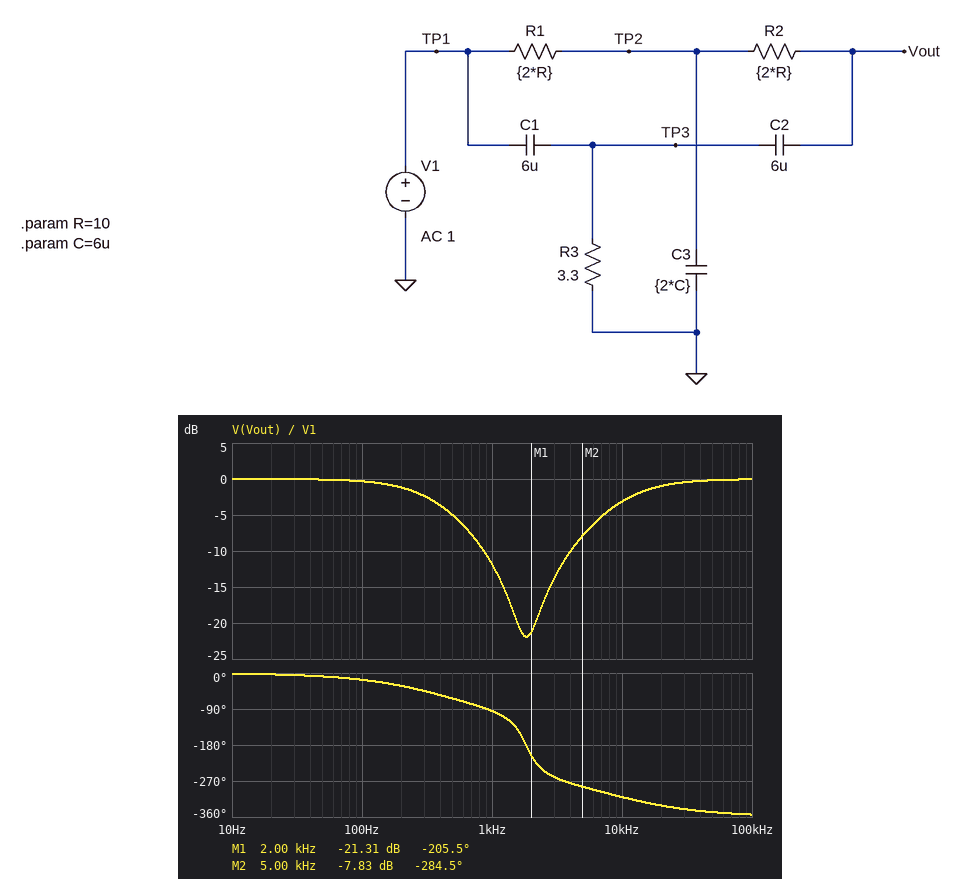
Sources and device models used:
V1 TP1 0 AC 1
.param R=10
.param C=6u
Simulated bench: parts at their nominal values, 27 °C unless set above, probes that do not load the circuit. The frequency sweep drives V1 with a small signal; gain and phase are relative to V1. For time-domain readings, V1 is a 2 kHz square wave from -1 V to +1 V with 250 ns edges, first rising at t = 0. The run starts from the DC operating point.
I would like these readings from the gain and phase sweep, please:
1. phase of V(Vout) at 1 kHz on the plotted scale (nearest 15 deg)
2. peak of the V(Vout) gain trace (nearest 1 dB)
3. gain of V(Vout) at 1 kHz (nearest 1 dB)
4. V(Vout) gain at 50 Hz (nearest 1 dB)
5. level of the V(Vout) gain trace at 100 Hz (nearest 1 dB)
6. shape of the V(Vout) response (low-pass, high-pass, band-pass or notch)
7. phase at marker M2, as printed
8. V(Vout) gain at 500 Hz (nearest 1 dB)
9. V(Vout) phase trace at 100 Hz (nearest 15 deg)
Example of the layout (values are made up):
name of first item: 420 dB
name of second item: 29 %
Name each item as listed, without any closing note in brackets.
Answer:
phase of V(Vout) at 1 kHz on the plotted scale: -90 deg
peak of the V(Vout) gain trace: 0 dB
gain of V(Vout) at 1 kHz: -12 dB
V(Vout) gain at 50 Hz: 0 dB
level of the V(Vout) gain trace at 100 Hz: 0 dB
shape of the V(Vout) response: notch
phase at marker M2, as printed: -284.5 deg
V(Vout) gain at 500 Hz: -5 dB
V(Vout) phase trace at 100 Hz: -15 deg
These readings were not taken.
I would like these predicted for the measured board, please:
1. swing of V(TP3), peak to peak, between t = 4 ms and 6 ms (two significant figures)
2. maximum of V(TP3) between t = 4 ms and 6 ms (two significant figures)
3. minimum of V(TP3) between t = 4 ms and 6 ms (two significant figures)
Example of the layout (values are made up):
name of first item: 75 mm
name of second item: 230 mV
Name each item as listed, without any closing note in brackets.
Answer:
swing of V(TP3), peak to peak, between t = 4 ms and 6 ms: 3.9 V
maximum of V(TP3) between t = 4 ms and 6 ms: 1.9 V
minimum of V(TP3) between t = 4 ms and 6 ms: -1.9 V
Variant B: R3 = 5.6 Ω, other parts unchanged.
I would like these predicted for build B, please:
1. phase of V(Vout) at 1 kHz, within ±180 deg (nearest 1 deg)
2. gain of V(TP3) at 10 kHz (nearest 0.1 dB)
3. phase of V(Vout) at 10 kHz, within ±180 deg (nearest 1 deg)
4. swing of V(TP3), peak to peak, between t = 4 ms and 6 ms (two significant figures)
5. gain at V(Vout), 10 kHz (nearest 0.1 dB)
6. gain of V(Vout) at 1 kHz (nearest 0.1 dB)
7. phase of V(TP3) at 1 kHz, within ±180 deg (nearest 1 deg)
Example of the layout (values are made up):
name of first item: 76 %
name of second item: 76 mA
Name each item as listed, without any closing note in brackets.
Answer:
phase of V(Vout) at 1 kHz, within ±180 deg: -94 deg
gain of V(TP3) at 10 kHz: -1.6 dB
phase of V(Vout) at 10 kHz, within ±180 deg: 38 deg
swing of V(TP3), peak to peak, between t = 4 ms and 6 ms: 3.8 V
gain at V(Vout), 10 kHz: -1.8 dB
gain of V(Vout) at 1 kHz: -13.6 dB
phase of V(TP3) at 1 kHz, within ±180 deg: 55 deg
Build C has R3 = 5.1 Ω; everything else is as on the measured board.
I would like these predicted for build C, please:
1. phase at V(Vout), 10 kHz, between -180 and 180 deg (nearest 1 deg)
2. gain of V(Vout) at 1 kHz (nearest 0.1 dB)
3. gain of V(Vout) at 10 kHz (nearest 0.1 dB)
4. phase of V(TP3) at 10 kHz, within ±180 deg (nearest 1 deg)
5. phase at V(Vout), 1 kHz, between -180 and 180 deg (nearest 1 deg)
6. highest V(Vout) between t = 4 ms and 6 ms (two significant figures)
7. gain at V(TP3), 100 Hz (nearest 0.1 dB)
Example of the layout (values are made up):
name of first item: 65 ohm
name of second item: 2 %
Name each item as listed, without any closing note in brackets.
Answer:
phase at V(Vout), 10 kHz, between -180 and 180 deg: 40 deg
gain of V(Vout) at 1 kHz: -13.2 dB
gain of V(Vout) at 10 kHz: -2.0 dB
phase of V(TP3) at 10 kHz, within ±180 deg: 32 deg
phase at V(Vout), 1 kHz, between -180 and 180 deg: -94 deg
highest V(Vout) between t = 4 ms and 6 ms: 1.8 V
gain at V(TP3), 100 Hz: -28.6 dB
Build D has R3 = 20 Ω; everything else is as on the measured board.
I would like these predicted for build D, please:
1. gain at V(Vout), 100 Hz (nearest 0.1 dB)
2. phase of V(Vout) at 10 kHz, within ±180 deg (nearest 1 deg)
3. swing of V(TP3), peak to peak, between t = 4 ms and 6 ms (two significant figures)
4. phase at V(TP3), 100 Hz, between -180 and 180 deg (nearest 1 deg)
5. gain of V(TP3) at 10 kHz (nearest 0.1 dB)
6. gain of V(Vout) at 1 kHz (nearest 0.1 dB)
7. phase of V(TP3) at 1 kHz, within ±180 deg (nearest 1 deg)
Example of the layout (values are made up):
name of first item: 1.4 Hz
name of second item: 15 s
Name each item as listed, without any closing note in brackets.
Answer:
gain at V(Vout), 100 Hz: -0.5 dB
phase of V(Vout) at 10 kHz, within ±180 deg: 22 deg
swing of V(TP3), peak to peak, between t = 4 ms and 6 ms: 3.4 V
phase at V(TP3), 100 Hz, between -180 and 180 deg: 73 deg
gain of V(TP3) at 10 kHz: -0.6 dB
gain of V(Vout) at 1 kHz: -17.7 dB
phase of V(TP3) at 1 kHz, within ±180 deg: 30 deg
